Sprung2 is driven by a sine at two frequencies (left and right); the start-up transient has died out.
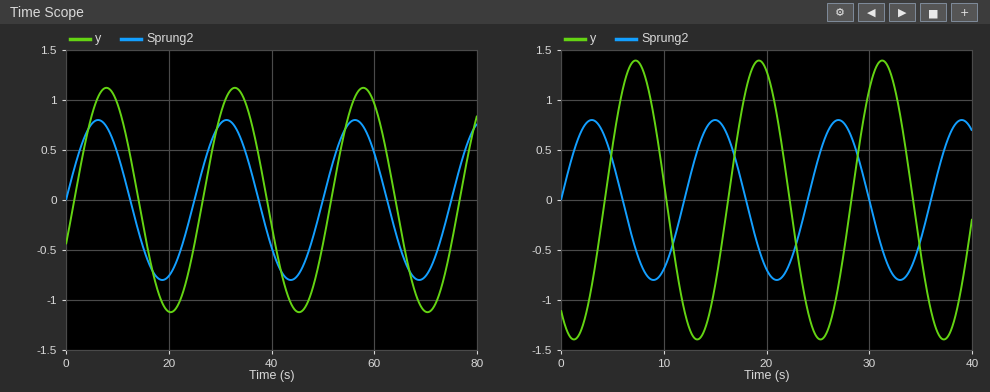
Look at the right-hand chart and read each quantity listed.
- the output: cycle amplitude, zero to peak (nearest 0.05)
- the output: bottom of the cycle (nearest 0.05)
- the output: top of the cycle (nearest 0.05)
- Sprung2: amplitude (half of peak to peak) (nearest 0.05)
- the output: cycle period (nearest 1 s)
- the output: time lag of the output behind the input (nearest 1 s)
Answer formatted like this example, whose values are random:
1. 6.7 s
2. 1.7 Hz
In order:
1. 1.40
2. -1.40
3. 1.40
4. 0.80
5. 12 s
6. 4 s
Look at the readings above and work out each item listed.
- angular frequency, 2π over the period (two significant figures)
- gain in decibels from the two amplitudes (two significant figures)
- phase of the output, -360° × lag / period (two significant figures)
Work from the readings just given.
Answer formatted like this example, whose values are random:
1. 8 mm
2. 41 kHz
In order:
1. 0.52 rad/s
2. 4.9 dB
3. -120°
